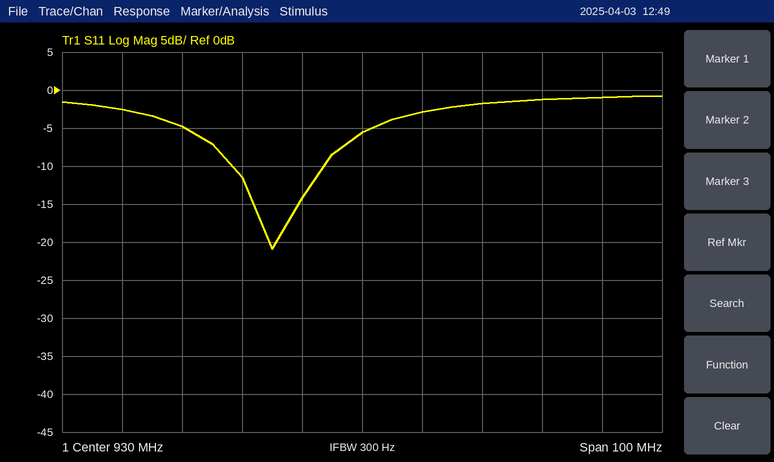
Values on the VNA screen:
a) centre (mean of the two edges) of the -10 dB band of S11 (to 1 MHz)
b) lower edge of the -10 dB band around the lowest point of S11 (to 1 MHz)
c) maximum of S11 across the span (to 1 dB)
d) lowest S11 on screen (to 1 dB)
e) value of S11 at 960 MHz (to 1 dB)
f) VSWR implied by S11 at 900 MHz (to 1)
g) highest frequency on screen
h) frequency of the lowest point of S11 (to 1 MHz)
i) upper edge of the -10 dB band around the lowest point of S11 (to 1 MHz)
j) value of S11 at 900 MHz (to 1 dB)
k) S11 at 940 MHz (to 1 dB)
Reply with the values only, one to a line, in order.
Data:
916 MHz
908 MHz
-1 dB
-21 dB
-1 dB
4
980 MHz
915 MHz
924 MHz
-5 dB
-3 dB
